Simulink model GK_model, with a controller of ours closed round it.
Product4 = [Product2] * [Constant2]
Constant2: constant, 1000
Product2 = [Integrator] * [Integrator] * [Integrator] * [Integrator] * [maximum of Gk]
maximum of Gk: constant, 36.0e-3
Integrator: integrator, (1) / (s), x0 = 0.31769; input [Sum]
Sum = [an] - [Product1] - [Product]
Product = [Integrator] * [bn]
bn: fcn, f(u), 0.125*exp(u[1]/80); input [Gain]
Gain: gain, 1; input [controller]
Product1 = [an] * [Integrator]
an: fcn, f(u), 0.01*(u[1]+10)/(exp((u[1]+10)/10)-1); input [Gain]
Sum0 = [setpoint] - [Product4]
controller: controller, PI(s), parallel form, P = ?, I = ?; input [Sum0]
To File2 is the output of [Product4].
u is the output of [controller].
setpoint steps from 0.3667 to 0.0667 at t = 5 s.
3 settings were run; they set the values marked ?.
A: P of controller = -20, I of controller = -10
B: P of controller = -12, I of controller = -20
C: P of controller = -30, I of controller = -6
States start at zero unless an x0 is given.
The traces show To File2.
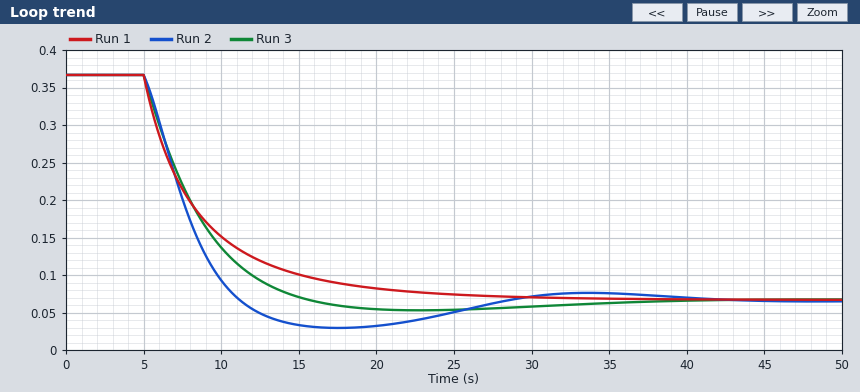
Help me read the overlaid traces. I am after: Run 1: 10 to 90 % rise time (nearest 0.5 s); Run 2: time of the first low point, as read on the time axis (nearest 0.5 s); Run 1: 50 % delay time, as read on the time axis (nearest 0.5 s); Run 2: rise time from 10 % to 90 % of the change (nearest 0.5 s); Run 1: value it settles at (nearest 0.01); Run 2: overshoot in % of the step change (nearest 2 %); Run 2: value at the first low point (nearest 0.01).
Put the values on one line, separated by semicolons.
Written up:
10.5 s; 17.5 s; 7.5 s; 4.5 s; 0.07; 12 %; 0.03
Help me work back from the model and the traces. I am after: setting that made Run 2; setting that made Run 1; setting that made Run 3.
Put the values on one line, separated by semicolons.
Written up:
B; C; A
